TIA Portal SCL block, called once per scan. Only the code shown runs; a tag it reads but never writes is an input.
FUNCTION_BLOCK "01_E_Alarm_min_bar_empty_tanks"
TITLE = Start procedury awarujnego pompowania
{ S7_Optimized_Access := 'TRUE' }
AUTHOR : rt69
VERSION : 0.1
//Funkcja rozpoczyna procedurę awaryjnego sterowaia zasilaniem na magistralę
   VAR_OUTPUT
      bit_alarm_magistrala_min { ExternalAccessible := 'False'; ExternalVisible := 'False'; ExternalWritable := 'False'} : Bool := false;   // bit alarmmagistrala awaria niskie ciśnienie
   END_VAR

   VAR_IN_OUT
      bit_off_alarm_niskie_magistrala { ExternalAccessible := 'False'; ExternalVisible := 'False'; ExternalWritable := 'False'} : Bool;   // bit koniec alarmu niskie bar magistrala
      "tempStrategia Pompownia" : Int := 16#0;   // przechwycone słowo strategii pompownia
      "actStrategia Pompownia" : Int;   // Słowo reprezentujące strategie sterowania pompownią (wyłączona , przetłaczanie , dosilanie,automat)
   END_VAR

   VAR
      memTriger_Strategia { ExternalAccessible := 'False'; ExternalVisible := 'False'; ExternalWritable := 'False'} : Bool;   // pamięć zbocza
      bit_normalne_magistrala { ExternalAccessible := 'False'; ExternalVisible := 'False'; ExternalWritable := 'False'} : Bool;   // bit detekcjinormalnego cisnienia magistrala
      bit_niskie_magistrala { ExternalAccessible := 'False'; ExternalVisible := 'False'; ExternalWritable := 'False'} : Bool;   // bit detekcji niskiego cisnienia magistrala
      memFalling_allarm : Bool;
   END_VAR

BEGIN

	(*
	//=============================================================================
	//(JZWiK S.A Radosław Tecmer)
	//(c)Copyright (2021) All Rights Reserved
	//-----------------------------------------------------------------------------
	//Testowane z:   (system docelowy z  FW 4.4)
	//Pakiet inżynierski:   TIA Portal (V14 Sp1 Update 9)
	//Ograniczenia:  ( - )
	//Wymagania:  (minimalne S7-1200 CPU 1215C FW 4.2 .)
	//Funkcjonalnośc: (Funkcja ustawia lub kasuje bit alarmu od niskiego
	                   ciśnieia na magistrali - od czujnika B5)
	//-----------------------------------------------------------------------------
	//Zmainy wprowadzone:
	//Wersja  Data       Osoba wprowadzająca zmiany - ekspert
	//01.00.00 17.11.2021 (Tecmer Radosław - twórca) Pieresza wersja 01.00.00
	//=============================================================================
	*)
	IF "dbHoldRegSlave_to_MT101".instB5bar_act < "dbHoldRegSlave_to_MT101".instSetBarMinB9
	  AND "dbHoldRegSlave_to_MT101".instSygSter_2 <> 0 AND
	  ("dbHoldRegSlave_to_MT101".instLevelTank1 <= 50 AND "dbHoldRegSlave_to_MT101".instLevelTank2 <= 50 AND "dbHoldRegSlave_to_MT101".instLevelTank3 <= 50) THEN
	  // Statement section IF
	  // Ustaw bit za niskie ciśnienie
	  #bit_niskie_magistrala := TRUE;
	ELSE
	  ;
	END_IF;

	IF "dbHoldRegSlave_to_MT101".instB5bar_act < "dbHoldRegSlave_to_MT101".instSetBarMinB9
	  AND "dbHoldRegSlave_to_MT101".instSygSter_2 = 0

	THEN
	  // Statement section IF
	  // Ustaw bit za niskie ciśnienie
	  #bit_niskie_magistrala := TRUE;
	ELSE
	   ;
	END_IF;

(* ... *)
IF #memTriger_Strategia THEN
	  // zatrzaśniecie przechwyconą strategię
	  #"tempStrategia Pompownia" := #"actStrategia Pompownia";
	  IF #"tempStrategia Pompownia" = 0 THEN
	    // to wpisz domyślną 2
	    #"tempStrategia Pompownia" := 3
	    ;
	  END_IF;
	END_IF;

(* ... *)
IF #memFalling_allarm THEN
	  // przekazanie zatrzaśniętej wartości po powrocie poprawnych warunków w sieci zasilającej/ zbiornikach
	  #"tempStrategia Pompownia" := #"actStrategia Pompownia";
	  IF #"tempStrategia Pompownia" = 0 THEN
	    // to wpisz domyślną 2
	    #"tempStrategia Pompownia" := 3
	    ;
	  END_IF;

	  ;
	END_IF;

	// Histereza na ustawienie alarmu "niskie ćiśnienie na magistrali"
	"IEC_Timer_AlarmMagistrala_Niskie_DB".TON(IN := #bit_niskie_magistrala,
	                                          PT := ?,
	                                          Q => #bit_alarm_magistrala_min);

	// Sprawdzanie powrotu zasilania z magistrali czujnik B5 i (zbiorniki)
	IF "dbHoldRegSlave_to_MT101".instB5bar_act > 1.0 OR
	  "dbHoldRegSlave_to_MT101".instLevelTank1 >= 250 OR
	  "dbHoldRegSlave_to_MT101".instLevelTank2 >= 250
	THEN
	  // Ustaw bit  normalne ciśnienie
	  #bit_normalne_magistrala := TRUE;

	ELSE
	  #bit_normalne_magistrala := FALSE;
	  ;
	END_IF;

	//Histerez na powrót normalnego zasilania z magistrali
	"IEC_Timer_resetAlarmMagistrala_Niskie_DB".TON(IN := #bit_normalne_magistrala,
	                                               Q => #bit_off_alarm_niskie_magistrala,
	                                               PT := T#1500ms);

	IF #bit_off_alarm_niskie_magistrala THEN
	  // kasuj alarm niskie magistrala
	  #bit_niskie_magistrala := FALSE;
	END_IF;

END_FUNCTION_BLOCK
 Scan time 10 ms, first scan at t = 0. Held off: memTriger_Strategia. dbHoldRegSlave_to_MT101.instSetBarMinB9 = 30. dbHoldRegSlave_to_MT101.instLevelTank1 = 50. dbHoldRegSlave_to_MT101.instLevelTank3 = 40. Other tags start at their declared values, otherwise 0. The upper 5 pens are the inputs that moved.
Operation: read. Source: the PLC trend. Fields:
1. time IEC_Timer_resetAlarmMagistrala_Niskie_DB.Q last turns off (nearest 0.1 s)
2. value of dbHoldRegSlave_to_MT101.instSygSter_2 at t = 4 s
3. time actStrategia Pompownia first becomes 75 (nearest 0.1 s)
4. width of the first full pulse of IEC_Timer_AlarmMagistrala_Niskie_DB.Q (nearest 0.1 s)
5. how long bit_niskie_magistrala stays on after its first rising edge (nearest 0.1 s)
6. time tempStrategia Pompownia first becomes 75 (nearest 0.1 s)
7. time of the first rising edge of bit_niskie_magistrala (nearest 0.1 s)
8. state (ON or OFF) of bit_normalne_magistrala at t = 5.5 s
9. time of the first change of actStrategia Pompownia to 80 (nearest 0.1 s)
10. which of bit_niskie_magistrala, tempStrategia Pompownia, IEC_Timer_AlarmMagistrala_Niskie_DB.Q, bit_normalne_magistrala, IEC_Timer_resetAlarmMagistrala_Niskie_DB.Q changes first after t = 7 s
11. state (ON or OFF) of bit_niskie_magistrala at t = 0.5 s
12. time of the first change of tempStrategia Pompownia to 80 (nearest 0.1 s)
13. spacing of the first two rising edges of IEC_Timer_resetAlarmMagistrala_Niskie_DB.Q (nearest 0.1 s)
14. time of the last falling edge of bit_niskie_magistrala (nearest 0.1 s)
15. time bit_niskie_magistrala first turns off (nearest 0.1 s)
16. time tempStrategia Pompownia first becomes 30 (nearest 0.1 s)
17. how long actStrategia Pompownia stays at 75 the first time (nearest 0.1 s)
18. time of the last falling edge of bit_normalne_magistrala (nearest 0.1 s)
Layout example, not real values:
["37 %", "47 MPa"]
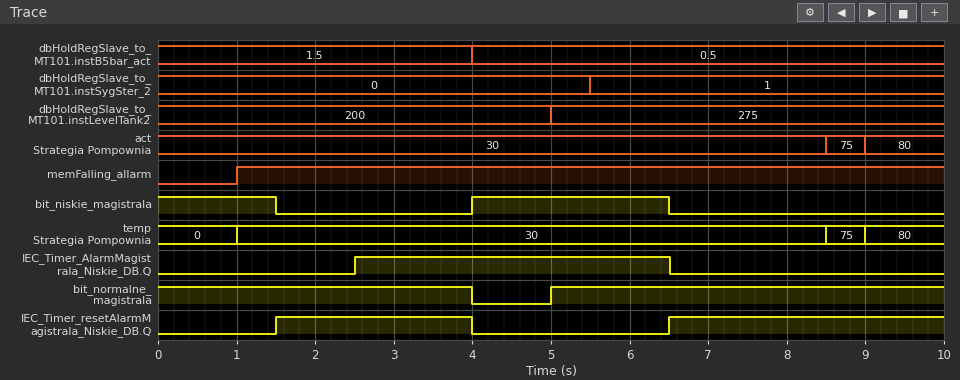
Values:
["4.0 s", "0", "8.5 s", "4.0 s", "2.5 s", "8.5 s", "4.0 s", "ON", "9.0 s", "tempStrategia Pompownia", "ON", "9.0 s", "5.0 s", "6.5 s", "1.5 s", "1.0 s", "0.5 s", "4.0 s"]
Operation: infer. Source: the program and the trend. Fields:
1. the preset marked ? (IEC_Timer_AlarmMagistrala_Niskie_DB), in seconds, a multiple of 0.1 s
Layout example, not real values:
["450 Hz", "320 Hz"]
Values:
["2.5 s"]
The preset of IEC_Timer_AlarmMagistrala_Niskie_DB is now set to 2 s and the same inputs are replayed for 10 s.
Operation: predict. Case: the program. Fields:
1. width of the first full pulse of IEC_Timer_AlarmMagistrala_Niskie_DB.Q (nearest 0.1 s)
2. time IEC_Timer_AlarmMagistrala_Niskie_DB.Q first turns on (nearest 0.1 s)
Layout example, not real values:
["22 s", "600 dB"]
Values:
["4.5 s", "2.0 s"]
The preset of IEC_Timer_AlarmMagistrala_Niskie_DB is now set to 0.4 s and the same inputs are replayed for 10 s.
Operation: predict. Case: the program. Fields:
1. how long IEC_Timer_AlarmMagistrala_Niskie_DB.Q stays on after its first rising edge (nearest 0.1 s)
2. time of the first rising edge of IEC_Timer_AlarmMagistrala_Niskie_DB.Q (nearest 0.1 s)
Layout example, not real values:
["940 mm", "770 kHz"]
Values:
["6.1 s", "0.4 s"]
